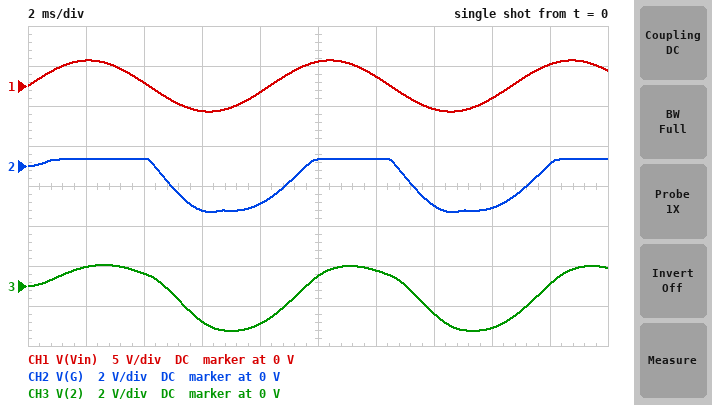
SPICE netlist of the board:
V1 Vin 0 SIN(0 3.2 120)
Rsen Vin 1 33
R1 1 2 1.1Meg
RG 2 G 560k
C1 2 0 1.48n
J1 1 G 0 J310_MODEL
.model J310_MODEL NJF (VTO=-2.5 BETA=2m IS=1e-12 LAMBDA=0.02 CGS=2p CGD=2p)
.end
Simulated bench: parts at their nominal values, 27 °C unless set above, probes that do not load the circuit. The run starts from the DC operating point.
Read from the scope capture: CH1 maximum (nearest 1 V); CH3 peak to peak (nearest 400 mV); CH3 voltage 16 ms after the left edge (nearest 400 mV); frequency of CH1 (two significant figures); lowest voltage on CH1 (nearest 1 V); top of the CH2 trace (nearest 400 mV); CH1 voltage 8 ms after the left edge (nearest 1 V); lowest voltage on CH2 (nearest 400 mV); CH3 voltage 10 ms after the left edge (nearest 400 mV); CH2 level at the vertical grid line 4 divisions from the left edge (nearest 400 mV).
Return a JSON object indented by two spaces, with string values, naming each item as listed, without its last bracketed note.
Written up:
{
  "CH1 maximum": "3 V",
  "CH3 peak to peak": "3.2 V",
  "CH3 voltage 16 ms after the left edge": "-2.0 V",
  "frequency of CH1": "120 Hz",
  "lowest voltage on CH1": "-3 V",
  "top of the CH2 trace": "400 mV",
  "CH1 voltage 8 ms after the left edge": "-1 V",
  "lowest voltage on CH2": "-2.4 V",
  "CH3 voltage 10 ms after the left edge": "400 mV",
  "CH2 level at the vertical grid line 4 divisions from the left edge": "-2.0 V"
}
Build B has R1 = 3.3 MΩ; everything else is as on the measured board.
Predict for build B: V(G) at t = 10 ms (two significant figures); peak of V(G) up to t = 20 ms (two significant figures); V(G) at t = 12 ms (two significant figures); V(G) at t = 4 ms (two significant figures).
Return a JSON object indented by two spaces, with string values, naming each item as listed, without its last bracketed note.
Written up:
{
  "V(G) at t = 10 ms": "-800 mV",
  "peak of V(G) up to t = 20 ms": "340 mV",
  "V(G) at t = 12 ms": "210 mV",
  "V(G) at t = 4 ms": "320 mV"
}
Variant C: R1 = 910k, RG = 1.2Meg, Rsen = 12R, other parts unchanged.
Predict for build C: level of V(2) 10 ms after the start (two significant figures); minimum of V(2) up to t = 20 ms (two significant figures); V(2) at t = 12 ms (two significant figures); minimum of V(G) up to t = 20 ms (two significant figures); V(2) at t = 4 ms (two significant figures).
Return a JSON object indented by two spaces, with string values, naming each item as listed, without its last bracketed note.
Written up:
{
  "level of V(2) 10 ms after the start": "840 mV",
  "minimum of V(2) up to t = 20 ms": "-2.5 V",
  "V(2) at t = 12 ms": "1.3 V",
  "minimum of V(G) up to t = 20 ms": "-2.7 V",
  "V(2) at t = 4 ms": "1.0 V"
}
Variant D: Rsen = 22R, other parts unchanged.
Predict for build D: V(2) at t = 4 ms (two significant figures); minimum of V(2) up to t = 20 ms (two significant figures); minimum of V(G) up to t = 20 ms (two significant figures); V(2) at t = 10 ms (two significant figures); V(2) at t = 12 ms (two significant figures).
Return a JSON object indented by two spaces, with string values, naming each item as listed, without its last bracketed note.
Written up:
{
  "V(2) at t = 4 ms": "650 mV",
  "minimum of V(2) up to t = 20 ms": "-2.4 V",
  "minimum of V(G) up to t = 20 ms": "-2.5 V",
  "V(2) at t = 10 ms": "520 mV",
  "V(2) at t = 12 ms": "820 mV"
}
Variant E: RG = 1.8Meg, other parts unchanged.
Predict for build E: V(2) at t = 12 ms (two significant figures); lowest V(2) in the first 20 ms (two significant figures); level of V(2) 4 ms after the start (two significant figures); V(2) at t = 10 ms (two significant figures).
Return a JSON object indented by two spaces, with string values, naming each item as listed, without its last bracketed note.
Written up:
{
  "V(2) at t = 12 ms": "1.2 V",
  "lowest V(2) in the first 20 ms": "-2.0 V",
  "level of V(2) 4 ms after the start": "1.0 V",
  "V(2) at t = 10 ms": "540 mV"
}
